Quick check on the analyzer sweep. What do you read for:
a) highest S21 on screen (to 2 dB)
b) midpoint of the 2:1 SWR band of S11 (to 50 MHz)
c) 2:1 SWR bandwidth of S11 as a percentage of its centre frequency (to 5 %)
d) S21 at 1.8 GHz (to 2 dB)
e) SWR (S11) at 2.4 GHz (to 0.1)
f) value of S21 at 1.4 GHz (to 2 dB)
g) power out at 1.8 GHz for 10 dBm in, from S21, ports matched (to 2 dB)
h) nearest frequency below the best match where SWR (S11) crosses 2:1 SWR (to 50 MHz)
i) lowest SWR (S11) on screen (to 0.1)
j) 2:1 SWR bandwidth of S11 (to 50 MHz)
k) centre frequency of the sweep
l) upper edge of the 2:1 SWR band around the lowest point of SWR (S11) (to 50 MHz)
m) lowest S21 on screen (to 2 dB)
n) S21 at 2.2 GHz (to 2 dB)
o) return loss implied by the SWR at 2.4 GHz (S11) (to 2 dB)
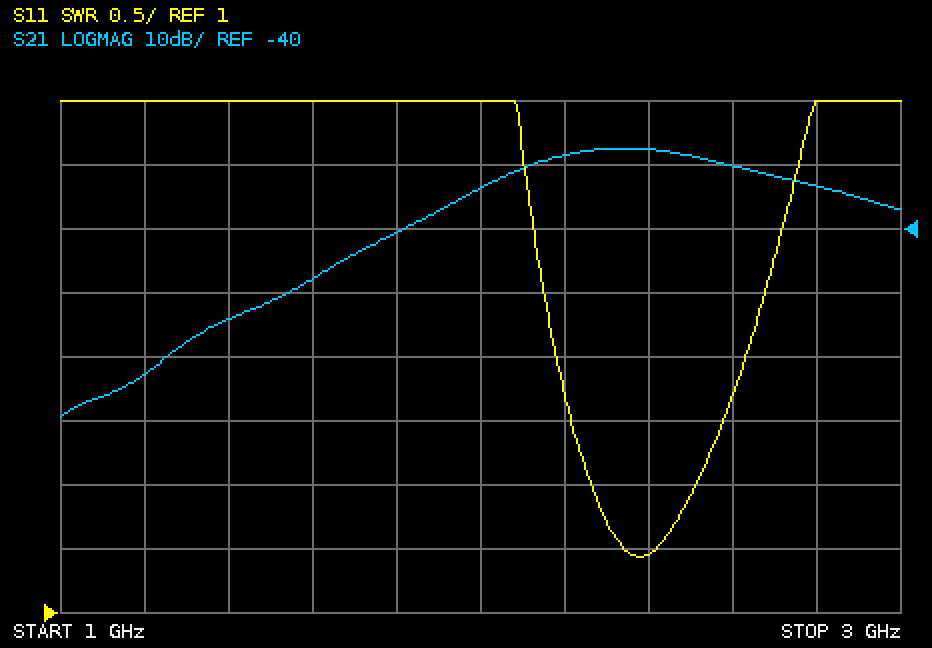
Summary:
-28 dB
2.40 GHz
10 %
-40 dB
1.5
-54 dB
-30 dBm
2.25 GHz
1.4
250 MHz
2 GHz
2.50 GHz
-70 dB
-28 dB
14 dB
